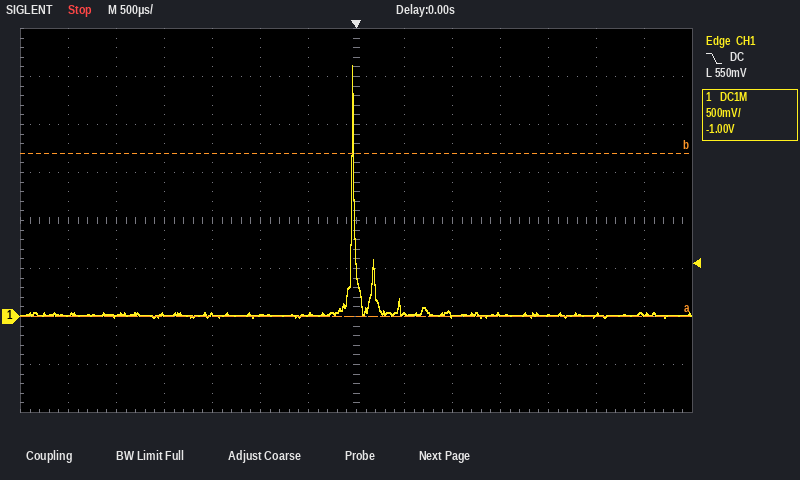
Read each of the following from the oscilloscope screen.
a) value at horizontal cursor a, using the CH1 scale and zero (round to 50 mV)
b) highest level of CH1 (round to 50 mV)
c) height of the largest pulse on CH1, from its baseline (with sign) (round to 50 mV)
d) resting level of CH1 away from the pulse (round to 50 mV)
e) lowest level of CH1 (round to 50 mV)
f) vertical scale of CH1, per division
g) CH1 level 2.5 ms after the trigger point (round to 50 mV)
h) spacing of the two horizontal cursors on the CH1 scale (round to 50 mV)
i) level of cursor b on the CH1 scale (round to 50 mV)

0 mV
2.60 V
+2.60 V
0 mV
0 mV
500 mV
0 mV
1.70 V
1.70 V
